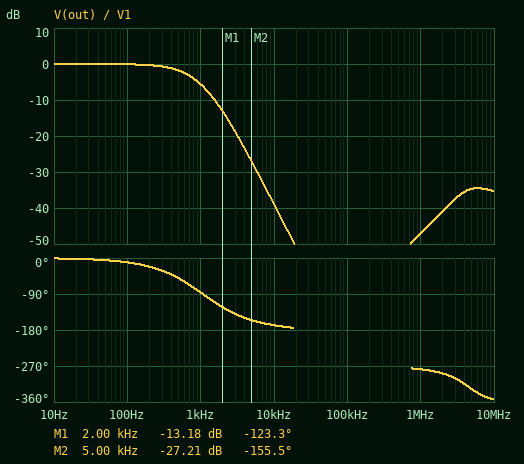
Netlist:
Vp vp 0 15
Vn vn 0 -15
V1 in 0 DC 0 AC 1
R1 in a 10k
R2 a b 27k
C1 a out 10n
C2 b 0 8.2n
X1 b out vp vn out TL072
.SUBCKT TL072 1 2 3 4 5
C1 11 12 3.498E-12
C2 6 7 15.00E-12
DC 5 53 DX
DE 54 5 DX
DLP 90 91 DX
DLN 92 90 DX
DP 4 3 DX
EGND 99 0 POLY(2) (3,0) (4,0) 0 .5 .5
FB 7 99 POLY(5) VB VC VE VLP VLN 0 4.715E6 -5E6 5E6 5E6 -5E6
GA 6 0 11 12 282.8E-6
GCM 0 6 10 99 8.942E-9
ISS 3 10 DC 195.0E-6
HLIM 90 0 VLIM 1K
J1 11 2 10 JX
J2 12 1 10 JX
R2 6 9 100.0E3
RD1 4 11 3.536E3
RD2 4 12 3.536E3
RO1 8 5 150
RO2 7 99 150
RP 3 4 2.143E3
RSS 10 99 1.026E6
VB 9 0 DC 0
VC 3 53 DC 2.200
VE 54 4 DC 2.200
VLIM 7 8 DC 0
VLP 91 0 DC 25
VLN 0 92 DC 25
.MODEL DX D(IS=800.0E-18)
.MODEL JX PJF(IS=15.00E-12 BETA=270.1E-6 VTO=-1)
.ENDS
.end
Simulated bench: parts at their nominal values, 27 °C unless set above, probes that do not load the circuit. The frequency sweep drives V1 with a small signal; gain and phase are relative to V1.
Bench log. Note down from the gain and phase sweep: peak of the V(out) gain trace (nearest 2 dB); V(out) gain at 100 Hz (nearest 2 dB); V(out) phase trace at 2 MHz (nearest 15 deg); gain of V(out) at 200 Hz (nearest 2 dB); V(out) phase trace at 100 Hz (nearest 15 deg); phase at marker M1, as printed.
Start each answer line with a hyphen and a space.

- 0 dB
- 0 dB
- -285 deg
- 0 dB
- -15 deg
- -123.3 deg
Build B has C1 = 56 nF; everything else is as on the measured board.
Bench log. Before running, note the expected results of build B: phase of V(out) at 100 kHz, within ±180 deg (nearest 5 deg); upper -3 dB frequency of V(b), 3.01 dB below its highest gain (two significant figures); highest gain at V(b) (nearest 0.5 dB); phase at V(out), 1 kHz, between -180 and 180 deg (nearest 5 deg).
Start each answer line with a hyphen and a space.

- 90 deg
- 540 Hz
- 2.0 dB
- -155 deg
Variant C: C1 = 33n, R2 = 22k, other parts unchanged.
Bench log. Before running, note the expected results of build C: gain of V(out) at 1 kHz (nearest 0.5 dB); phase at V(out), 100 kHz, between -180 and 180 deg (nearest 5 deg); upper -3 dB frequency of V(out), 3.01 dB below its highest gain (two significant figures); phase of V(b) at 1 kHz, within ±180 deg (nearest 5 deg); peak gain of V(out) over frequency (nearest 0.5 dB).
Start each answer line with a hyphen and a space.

- -6.5 dB
- 95 deg
- 750 Hz
- -130 deg
- 1.0 dB
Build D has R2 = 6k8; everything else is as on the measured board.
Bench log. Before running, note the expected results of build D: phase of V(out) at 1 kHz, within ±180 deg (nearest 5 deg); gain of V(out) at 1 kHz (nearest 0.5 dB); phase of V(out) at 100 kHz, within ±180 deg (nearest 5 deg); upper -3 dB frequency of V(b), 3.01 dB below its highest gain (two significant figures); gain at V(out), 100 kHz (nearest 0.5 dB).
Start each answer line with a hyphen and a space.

- -50 deg
- -1.5 dB
- 135 deg
- 1.5 kHz
- -64.0 dB
